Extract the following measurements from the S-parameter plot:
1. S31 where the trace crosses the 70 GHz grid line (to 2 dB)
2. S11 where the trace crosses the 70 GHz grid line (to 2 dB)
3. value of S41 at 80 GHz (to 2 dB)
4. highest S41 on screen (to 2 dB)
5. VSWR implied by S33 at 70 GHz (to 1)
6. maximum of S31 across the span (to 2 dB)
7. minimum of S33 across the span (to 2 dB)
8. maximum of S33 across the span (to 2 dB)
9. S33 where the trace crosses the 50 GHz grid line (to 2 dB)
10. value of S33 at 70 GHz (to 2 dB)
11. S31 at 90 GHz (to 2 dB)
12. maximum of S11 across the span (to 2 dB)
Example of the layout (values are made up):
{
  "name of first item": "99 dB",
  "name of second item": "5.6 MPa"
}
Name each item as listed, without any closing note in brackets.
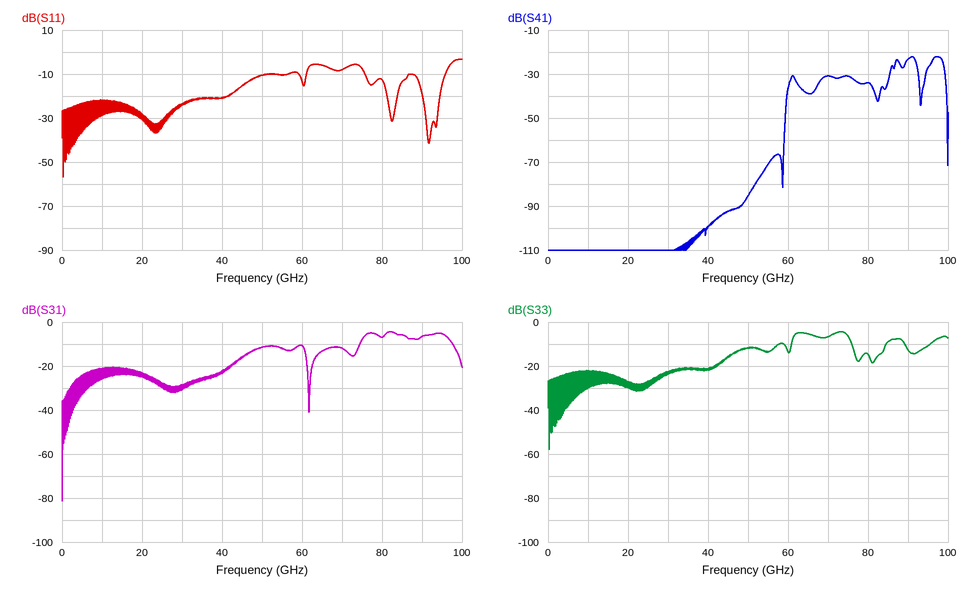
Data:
{
  "S31 where the trace crosses the 70 GHz grid line": "-12 dB",
  "S11 where the trace crosses the 70 GHz grid line": "-8 dB",
  "value of S41 at 80 GHz": "-34 dB",
  "highest S41 on screen": "-22 dB",
  "VSWR implied by S33 at 70 GHz": "3",
  "maximum of S31 across the span": "-4 dB",
  "minimum of S33 across the span": "-58 dB",
  "maximum of S33 across the span": "-4 dB",
  "S33 where the trace crosses the 50 GHz grid line": "-12 dB",
  "value of S33 at 70 GHz": "-6 dB",
  "S31 at 90 GHz": "-6 dB",
  "maximum of S11 across the span": "-4 dB"
}
